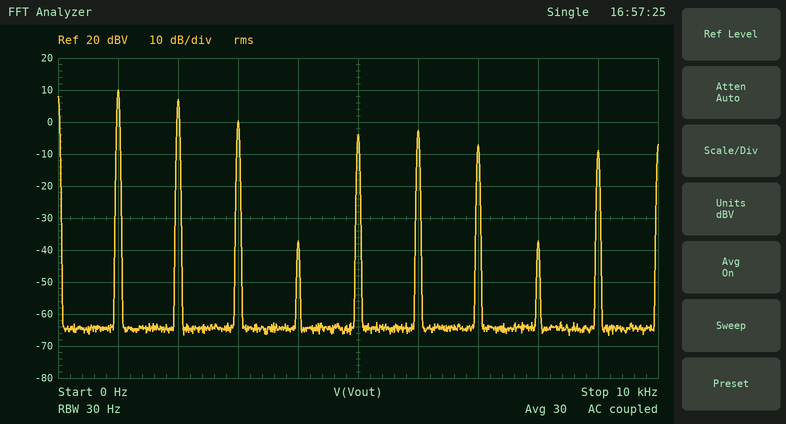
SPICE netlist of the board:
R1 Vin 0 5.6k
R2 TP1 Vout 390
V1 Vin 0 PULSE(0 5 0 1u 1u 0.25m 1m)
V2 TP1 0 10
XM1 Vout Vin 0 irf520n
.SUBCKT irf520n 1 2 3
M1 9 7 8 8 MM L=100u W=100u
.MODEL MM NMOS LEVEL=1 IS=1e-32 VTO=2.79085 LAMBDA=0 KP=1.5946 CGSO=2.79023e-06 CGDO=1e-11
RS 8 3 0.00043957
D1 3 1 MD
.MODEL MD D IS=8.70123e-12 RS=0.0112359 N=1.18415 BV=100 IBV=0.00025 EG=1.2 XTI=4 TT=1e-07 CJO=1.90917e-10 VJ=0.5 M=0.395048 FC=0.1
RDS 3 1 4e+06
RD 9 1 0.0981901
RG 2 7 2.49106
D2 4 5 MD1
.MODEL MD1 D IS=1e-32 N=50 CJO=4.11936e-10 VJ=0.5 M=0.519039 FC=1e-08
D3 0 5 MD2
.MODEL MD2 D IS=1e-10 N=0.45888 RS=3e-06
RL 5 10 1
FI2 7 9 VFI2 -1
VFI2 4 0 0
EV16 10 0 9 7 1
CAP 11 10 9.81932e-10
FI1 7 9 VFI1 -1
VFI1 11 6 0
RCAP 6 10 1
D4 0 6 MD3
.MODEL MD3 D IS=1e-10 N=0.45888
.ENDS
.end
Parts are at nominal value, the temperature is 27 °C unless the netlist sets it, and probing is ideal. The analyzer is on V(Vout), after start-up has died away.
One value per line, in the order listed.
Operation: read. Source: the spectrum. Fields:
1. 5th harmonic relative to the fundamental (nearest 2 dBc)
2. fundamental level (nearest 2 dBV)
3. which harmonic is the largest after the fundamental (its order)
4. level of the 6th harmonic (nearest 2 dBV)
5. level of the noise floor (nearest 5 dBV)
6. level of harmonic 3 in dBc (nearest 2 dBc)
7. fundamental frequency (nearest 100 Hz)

-14 dBc
10 dBV
2
-2 dBV
-65 dBV
-10 dBc
1.0 kHz
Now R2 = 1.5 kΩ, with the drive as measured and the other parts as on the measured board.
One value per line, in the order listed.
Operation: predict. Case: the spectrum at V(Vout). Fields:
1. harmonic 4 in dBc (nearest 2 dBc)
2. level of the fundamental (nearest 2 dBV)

-44 dBc
10 dBV
